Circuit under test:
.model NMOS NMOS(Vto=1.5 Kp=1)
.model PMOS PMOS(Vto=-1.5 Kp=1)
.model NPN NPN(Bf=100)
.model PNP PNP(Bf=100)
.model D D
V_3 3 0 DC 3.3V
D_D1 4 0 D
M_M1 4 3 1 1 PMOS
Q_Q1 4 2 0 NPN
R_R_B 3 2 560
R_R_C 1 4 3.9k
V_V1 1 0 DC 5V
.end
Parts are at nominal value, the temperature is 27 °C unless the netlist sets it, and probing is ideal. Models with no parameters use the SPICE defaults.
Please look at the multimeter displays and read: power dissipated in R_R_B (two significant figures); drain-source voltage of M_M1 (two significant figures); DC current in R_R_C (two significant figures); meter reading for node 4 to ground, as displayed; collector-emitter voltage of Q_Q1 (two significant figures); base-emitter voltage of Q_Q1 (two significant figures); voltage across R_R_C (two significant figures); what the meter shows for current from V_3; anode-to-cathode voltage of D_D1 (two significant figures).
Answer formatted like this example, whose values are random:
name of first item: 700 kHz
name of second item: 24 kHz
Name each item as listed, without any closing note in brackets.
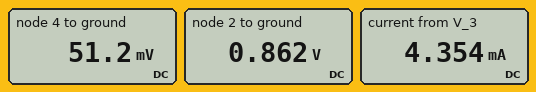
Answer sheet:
power dissipated in R_R_B: 11 mW
drain-source voltage of M_M1: -4.9 V
DC current in R_R_C: 1.3 mA
meter reading for node 4 to ground, as displayed: 51.2 mV
collector-emitter voltage of Q_Q1: 51 mV
base-emitter voltage of Q_Q1: 860 mV
voltage across R_R_C: 4.9 V
what the meter shows for current from V_3: 4.354 mA
anode-to-cathode voltage of D_D1: 51 mV
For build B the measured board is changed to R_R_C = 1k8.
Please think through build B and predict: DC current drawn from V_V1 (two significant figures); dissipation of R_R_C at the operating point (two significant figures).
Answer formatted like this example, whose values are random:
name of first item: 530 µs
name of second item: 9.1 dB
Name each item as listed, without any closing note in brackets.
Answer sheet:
DC current drawn from V_V1: 23 mA
dissipation of R_R_C at the operating point: 14 mW
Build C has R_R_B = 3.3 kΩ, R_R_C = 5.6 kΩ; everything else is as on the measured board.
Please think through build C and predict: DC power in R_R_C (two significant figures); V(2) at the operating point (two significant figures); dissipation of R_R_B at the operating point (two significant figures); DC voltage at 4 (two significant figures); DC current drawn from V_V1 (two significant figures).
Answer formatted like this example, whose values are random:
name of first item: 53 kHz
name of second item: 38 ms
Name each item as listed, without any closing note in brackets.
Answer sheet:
DC power in R_R_C: 4.3 mW
V(2) at the operating point: 850 mV
dissipation of R_R_B at the operating point: 1.8 mW
DC voltage at 4: 97 mV
DC current drawn from V_V1: 21 mA
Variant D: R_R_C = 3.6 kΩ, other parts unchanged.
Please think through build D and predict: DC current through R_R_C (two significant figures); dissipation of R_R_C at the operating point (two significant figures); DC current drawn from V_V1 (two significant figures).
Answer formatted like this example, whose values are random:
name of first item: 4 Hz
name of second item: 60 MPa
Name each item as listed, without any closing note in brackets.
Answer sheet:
DC current through R_R_C: 1.4 mA
dissipation of R_R_C at the operating point: 6.8 mW
DC current drawn from V_V1: 21 mA
